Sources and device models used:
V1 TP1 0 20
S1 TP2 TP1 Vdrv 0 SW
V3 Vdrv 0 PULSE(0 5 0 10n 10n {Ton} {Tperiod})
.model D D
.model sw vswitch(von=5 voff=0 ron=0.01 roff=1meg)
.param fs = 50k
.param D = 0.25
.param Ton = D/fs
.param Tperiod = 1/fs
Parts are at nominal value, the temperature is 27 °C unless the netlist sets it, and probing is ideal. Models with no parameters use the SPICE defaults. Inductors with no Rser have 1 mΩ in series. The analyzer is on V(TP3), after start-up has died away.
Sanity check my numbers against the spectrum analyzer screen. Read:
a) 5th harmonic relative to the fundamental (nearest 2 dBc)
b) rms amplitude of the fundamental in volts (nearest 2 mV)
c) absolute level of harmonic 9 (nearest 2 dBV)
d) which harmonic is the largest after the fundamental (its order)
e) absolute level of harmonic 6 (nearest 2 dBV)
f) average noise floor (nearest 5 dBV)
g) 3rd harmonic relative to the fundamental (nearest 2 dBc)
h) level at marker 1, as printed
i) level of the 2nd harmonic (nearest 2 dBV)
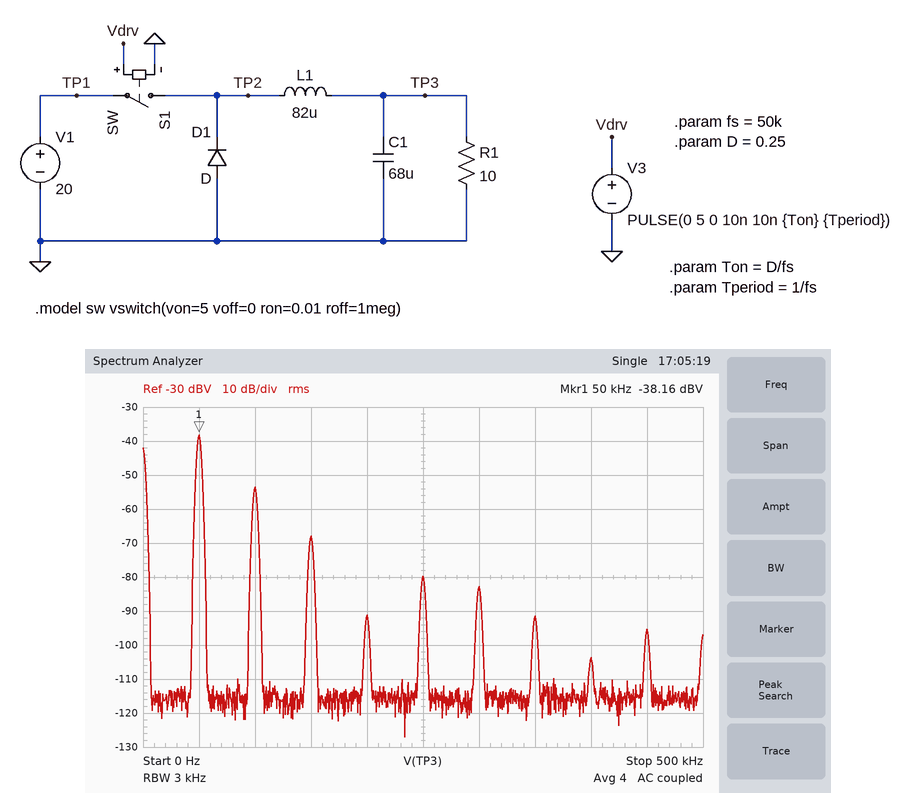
-42 dBc
12 mV
-96 dBV
2
-82 dBV
-115 dBV
-30 dBc
-38.16 dBV
-54 dBV
